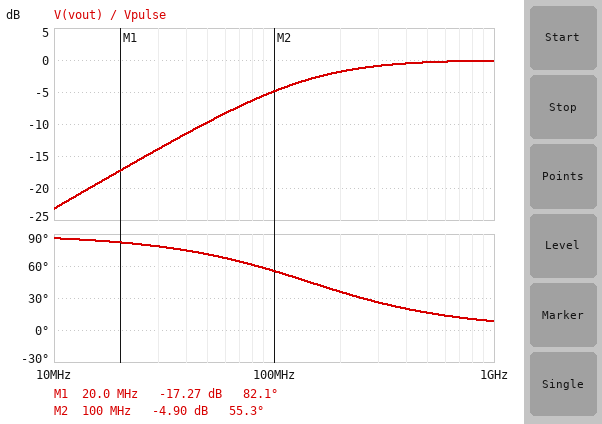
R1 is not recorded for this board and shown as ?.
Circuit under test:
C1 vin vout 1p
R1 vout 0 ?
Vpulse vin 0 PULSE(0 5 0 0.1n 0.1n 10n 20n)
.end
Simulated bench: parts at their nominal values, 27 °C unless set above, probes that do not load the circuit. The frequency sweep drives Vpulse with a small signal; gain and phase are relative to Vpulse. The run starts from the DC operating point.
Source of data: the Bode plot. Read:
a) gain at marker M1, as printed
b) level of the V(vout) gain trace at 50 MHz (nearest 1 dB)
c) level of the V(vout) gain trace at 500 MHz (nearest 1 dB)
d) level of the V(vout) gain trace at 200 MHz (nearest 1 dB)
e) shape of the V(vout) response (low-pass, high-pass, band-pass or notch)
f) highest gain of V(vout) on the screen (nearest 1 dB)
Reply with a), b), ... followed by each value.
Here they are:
a) -17.27 dB
b) -10 dB
c) 0 dB
d) -2 dB
e) high-pass
f) 0 dB
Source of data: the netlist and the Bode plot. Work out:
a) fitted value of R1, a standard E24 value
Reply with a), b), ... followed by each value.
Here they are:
a) 1.1 kΩ
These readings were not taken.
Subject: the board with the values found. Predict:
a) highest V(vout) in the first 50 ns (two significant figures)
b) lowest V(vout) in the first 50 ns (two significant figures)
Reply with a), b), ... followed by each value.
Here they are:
a) 4.8 V
b) -4.8 V
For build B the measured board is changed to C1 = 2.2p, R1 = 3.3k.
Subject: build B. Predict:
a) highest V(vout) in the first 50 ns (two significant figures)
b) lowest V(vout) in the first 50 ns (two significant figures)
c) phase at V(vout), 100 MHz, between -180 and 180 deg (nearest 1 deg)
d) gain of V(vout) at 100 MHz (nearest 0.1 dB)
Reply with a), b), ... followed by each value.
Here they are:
a) 5.0 V
b) -4.0 V
c) 12 deg
d) -0.2 dB
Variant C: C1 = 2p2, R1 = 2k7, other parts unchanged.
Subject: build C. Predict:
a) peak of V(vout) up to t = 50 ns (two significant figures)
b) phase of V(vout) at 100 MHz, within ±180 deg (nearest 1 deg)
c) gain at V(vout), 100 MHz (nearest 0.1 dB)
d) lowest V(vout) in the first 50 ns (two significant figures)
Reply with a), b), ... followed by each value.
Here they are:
a) 5.0 V
b) 15 deg
c) -0.3 dB
d) -4.2 V
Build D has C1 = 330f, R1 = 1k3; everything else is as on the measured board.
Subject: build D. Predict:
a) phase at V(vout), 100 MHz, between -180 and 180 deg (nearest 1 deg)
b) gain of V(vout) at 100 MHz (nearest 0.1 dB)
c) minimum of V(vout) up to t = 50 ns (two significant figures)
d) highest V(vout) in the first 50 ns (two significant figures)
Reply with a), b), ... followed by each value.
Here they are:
a) 75 deg
b) -11.7 dB
c) -4.5 V
d) 4.5 V
